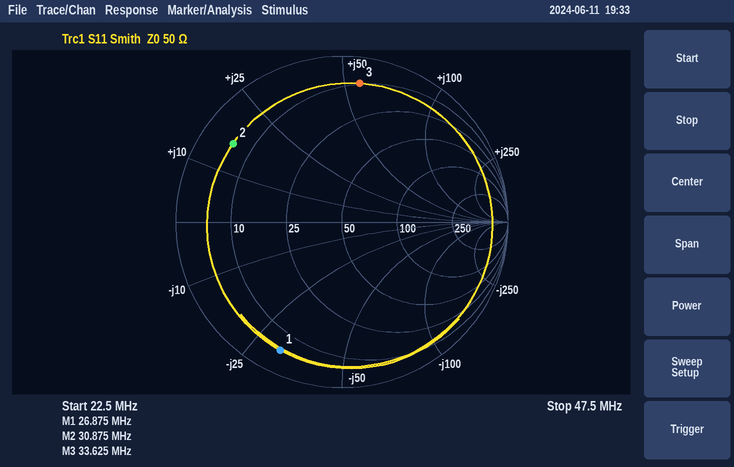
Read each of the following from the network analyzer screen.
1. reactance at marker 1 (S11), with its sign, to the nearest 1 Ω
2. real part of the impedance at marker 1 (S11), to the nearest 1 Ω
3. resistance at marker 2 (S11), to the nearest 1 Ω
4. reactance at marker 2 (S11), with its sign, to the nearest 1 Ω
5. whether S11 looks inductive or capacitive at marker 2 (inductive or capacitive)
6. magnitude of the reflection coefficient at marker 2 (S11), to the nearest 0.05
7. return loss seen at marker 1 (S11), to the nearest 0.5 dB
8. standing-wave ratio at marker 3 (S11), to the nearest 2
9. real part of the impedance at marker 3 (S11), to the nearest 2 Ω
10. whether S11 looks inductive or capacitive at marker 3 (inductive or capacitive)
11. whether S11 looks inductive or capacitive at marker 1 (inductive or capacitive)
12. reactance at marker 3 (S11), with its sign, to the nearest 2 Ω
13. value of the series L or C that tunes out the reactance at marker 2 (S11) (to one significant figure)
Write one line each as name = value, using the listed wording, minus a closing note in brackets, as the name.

reactance at marker 1 (S11), with its sign, to the nearest 1 Ω = -31 Ω
real part of the impedance at marker 1 (S11), to the nearest 1 Ω = 5 Ω
resistance at marker 2 (S11), to the nearest 1 Ω = 6 Ω
reactance at marker 2 (S11), with its sign, to the nearest 1 Ω = +16 Ω
whether S11 looks inductive or capacitive at marker 2 = inductive
magnitude of the reflection coefficient at marker 2 (S11), to the nearest 0.05 = 0.80
return loss seen at marker 1 (S11), to the nearest 0.5 dB = 1.5 dB
standing-wave ratio at marker 3 (S11), to the nearest 2 = 12
real part of the impedance at marker 3 (S11), to the nearest 2 Ω = 10 Ω
whether S11 looks inductive or capacitive at marker 3 = inductive
whether S11 looks inductive or capacitive at marker 1 = capacitive
reactance at marker 3 (S11), with its sign, to the nearest 2 Ω = +56 Ω
value of the series L or C that tunes out the reactance at marker 2 (S11) = 300 pF
